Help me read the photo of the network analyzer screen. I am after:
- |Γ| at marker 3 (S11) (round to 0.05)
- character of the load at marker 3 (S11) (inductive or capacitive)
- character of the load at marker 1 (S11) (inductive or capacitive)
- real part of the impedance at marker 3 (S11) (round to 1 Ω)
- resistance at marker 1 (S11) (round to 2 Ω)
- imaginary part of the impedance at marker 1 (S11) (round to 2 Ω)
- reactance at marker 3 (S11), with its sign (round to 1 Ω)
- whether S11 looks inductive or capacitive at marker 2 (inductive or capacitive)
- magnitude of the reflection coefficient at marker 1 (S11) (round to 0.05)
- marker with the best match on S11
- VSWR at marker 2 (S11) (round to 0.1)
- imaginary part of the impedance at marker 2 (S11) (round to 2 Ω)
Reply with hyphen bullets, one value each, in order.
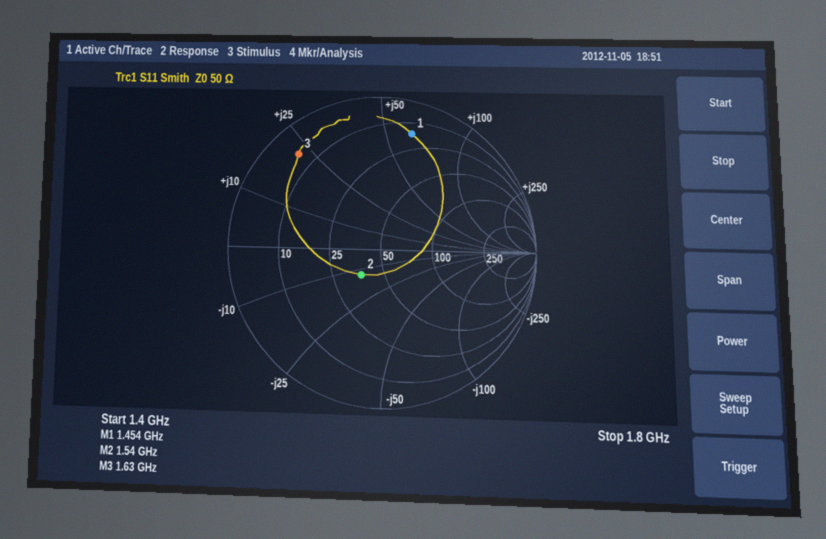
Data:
- 0.80
- inductive
- inductive
- 6 Ω
- 16 Ω
- +62 Ω
- +22 Ω
- capacitive
- 0.80
- marker 2
- 1.5
- -12 Ω
